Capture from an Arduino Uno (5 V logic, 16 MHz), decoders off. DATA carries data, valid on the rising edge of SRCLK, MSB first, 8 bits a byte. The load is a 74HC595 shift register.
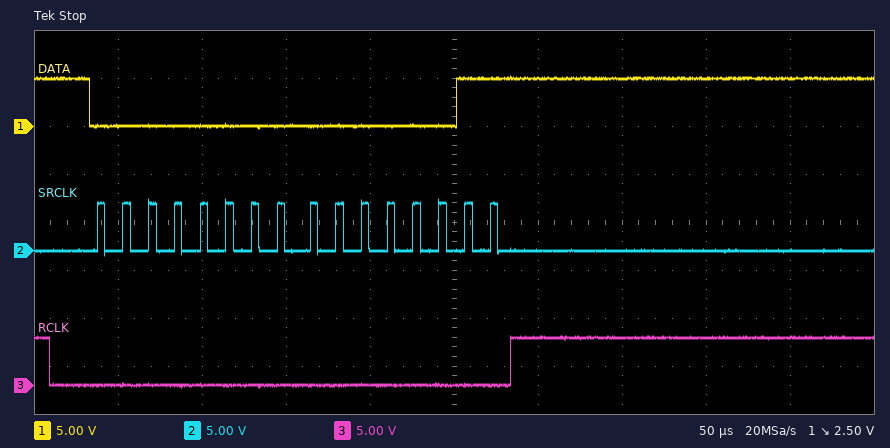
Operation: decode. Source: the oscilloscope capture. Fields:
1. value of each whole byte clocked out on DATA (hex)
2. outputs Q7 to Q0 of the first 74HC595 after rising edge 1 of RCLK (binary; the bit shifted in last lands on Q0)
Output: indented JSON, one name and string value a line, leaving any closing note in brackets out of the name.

{
  "value of each whole byte clocked out on DATA": "0x00 0x03",
  "outputs Q7 to Q0 of the first 74HC595 after rising edge 1 of RCLK": "00000011"
}
